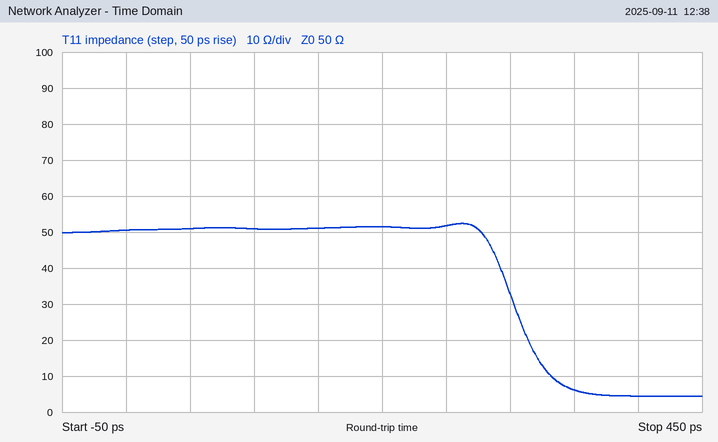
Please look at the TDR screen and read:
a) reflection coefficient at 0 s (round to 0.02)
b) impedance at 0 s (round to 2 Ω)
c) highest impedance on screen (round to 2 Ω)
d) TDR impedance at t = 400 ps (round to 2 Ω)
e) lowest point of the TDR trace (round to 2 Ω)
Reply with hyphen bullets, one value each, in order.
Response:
- 0.00
- 50 Ω
- 52 Ω
- 4 Ω
- 4 Ω
